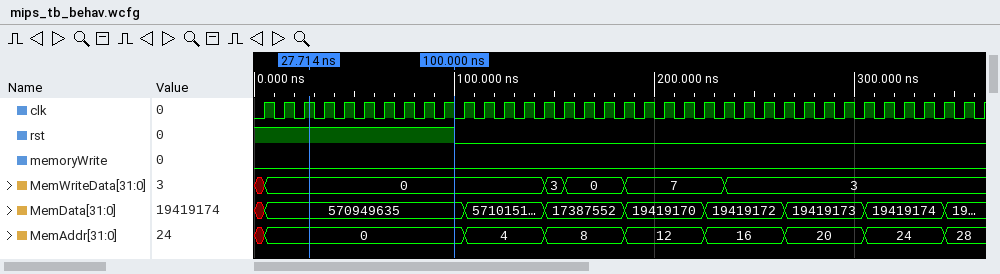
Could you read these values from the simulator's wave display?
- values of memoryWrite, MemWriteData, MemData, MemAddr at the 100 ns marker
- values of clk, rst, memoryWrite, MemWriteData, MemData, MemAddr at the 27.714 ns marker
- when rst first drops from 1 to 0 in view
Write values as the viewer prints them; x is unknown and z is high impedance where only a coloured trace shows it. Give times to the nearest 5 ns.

memoryWrite=0, MemWriteData=0, MemData=570949635, MemAddr=0
clk=1, rst=1, memoryWrite=0, MemWriteData=0, MemData=570949635, MemAddr=0
100 ns
